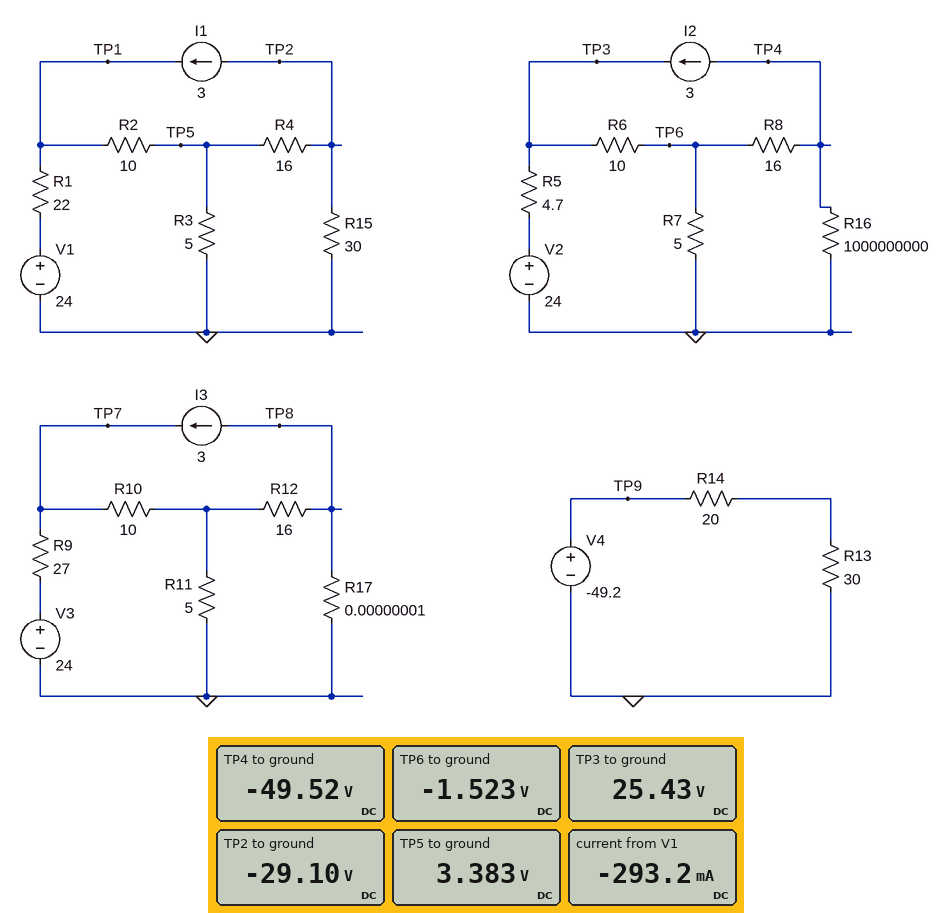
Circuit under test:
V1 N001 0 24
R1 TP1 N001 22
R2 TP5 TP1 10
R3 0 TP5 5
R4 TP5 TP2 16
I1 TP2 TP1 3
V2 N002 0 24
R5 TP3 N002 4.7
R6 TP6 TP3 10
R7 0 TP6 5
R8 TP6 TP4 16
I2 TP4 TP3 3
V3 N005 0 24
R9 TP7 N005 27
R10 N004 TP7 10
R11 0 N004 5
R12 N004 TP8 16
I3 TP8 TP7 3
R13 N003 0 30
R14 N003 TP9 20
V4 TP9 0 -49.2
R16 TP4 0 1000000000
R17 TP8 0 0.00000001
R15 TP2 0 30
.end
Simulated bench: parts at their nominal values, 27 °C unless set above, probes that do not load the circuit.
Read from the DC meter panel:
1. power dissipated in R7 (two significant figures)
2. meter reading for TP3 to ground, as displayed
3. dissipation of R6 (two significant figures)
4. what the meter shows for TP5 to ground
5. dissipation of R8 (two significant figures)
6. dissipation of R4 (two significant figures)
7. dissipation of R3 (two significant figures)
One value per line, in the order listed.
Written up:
460 mW
25.43 V
73 W
3.383 V
140 W
66 W
2.3 W
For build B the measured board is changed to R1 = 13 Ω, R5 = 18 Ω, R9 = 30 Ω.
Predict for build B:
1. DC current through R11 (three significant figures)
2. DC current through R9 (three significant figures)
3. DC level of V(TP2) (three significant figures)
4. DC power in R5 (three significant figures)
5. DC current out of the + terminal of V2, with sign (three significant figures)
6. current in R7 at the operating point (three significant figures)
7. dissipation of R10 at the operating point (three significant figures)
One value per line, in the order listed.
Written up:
1.98 A
398 mA
-29.4 V
595 mW
-182 mA
182 mA
67.7 W
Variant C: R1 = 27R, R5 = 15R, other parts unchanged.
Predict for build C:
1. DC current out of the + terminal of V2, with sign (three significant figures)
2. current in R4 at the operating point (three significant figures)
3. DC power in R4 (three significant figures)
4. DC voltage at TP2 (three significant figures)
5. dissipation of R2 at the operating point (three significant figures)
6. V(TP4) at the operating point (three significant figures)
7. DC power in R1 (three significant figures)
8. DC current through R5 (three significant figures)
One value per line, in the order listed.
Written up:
-200 mA
2.03 A
66.2 W
-29.0 V
75.2 W
-49.0 V
1.80 W
200 mA
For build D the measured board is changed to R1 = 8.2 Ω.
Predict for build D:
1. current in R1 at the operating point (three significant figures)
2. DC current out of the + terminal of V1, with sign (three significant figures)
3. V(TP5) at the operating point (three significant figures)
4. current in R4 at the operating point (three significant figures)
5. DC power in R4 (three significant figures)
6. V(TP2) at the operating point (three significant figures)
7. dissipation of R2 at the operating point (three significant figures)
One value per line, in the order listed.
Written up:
471 mA
-471 mA
2.58 V
2.01 A
64.8 W
-29.6 V
63.9 W
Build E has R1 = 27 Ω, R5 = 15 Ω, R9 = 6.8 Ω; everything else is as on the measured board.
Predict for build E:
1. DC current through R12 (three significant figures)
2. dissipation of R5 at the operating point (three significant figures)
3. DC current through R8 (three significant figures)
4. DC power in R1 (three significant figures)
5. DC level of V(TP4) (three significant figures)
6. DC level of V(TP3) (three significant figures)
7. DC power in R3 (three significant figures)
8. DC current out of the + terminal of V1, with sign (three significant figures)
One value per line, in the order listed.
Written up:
513 mA
600 mW
3.00 A
1.80 W
-49.0 V
27.0 V
2.51 W
-258 mA
